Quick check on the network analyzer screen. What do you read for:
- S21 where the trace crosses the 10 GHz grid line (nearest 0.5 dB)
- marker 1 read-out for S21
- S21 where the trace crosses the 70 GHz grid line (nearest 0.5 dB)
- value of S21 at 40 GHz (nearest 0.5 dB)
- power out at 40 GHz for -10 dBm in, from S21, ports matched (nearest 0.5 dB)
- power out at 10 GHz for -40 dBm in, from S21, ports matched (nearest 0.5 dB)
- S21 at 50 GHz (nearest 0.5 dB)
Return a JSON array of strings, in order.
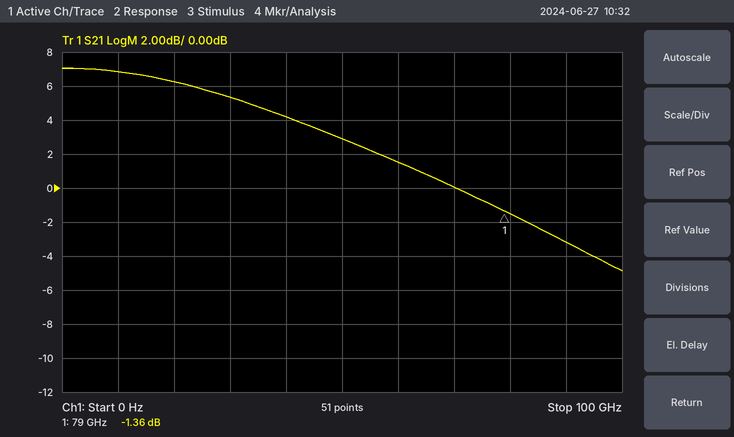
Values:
["7.0 dB", "-1.36 dB", "0.0 dB", "4.0 dB", "-6.0 dBm", "-33.0 dBm", "3.0 dB"]
